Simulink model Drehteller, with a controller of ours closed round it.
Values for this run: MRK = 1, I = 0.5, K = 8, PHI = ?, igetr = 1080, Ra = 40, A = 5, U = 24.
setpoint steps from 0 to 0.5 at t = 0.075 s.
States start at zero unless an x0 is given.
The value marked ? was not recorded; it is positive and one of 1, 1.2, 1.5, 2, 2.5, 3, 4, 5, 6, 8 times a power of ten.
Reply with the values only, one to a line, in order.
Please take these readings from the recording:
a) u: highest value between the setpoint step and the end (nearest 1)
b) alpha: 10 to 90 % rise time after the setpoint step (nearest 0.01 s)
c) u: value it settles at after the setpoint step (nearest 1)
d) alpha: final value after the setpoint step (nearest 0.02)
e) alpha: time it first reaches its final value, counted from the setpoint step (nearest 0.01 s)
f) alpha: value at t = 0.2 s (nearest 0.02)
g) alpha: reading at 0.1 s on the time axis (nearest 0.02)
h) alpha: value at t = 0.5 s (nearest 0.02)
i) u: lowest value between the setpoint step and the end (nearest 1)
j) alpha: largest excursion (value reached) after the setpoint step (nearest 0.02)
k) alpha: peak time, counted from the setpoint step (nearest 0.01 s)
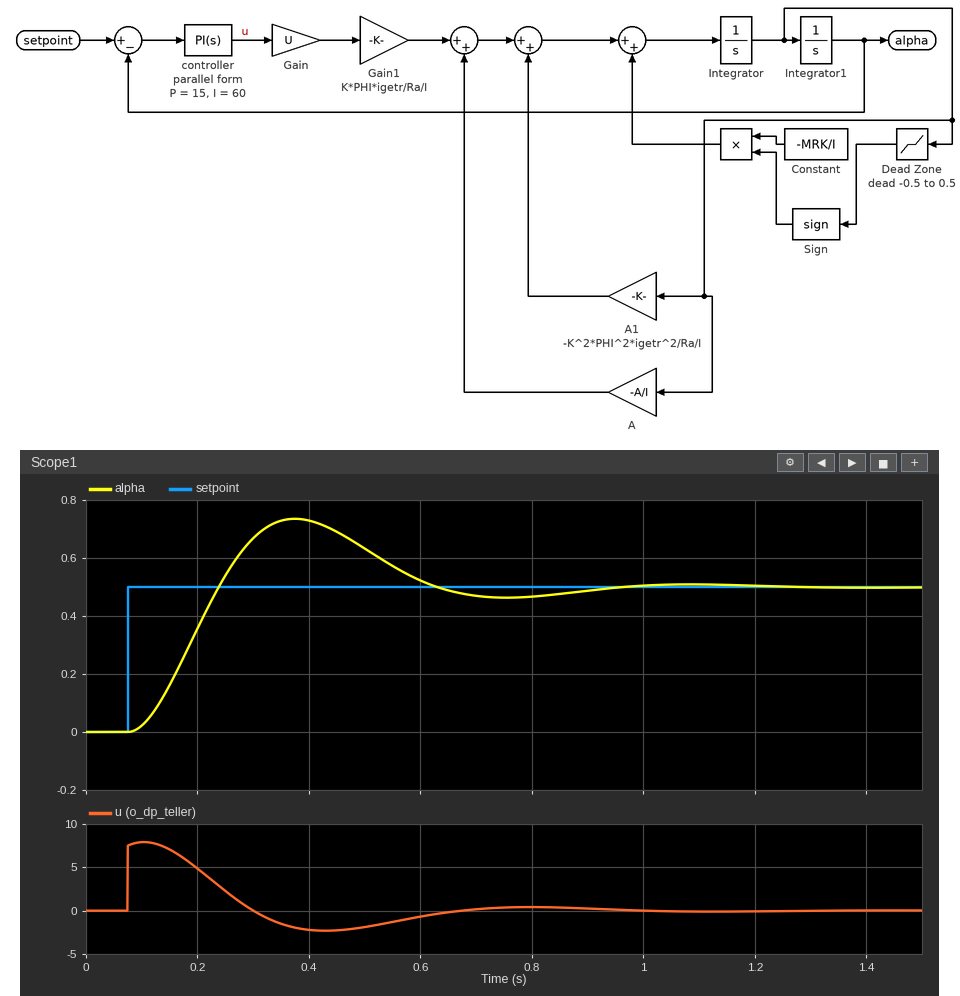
8
0.11 s
0
0.50
0.16 s
0.36
0.02
0.64
-2
0.74
0.30 s
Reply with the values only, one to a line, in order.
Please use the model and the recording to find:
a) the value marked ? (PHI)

0.001
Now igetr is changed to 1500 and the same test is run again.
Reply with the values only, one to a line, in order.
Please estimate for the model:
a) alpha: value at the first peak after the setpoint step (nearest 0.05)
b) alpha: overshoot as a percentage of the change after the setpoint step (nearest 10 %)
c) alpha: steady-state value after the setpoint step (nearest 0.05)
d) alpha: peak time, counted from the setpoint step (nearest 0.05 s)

0.70
40 %
0.50
0.25 s
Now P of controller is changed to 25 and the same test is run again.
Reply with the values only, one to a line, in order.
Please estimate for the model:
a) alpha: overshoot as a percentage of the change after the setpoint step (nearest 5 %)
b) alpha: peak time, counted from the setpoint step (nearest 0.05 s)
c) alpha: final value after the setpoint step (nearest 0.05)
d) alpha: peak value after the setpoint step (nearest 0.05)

40 %
0.20 s
0.50
0.70
